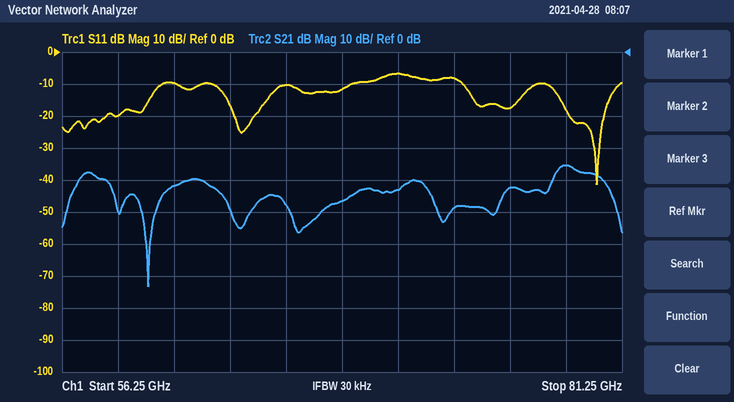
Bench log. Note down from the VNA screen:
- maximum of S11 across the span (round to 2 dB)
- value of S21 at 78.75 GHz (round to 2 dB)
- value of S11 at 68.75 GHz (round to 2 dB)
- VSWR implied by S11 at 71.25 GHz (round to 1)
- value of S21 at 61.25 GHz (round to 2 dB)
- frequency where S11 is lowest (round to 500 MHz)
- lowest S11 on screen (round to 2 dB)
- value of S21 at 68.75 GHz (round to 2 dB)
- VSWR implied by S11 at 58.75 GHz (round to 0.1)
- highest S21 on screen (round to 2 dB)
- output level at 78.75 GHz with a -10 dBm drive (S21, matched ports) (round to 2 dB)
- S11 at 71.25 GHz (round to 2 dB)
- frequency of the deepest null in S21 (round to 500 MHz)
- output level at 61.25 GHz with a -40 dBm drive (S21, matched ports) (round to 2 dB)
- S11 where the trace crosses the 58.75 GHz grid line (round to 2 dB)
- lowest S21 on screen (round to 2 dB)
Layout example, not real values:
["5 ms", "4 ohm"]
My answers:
["-6 dB", "-36 dB", "-12 dB", "3", "-42 dB", "80.0 GHz", "-42 dB", "-46 dB", "1.2", "-36 dB", "-46 dBm", "-6 dB", "60.0 GHz", "-82 dBm", "-20 dB", "-74 dB"]
